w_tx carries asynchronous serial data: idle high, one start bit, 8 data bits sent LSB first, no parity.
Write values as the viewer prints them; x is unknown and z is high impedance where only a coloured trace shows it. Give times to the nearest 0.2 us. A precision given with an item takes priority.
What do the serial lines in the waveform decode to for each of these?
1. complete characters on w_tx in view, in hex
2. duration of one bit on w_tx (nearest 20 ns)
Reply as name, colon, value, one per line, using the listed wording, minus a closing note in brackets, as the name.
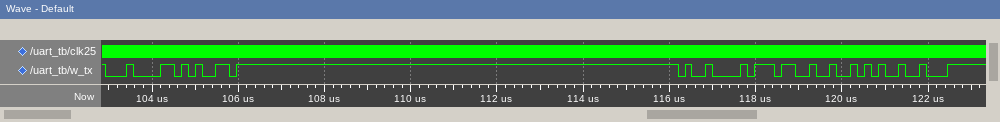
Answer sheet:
complete characters on w_tx in view, in hex: 84, 65, 09, 37, 52, 12
duration of one bit on w_tx: 160 ns
